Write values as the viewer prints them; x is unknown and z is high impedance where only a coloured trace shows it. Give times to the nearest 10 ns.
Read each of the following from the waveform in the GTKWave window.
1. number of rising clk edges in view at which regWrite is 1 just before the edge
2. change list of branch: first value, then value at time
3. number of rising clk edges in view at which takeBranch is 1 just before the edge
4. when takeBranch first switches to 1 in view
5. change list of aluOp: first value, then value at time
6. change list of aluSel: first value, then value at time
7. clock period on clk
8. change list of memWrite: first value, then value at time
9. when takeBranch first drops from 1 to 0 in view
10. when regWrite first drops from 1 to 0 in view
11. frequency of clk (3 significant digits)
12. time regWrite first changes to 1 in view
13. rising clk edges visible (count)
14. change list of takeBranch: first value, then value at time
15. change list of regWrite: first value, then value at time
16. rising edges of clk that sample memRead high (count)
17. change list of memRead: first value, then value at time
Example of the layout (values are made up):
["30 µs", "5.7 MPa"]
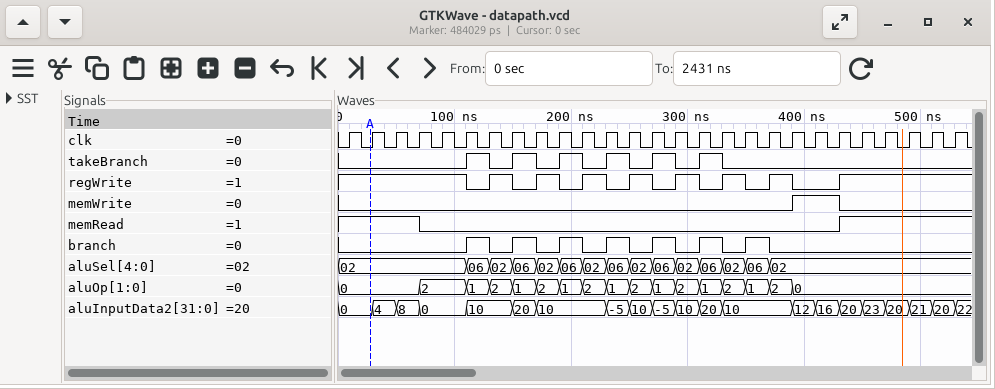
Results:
["18", "0, 1 at 110 ns, 0 at 130 ns, 1 at 150 ns, 0 at 170 ns, 1 at 190 ns, 0 at 210 ns, 1 at 230 ns, 0 at 250 ns, 1 at 270 ns, 0 at 290 ns, 1 at 310 ns, 0 at 330 ns, 1 at 350 ns, 0 at 370 ns", "6", "110 ns", "0, 2 at 70 ns, 1 at 110 ns, 2 at 130 ns, 1 at 150 ns, 2 at 170 ns, 1 at 190 ns, 2 at 210 ns, 1 at 230 ns, 2 at 250 ns, 1 at 270 ns, 2 at 290 ns, 1 at 310 ns, 2 at 330 ns, 1 at 350 ns, 2 at 370 ns, 0 at 390 ns", "02, 06 at 110 ns, 02 at 130 ns, 06 at 150 ns, 02 at 170 ns, 06 at 190 ns, 02 at 210 ns, 06 at 230 ns, 02 at 250 ns, 06 at 270 ns, 02 at 290 ns, 06 at 310 ns, 02 at 330 ns, 06 at 350 ns, 02 at 370 ns", "20 ns", "0, 1 at 390 ns, 0 at 430 ns", "130 ns", "110 ns", "50.0 MHz", "130 ns", "27", "0, 1 at 110 ns, 0 at 130 ns, 1 at 150 ns, 0 at 170 ns, 1 at 190 ns, 0 at 210 ns, 1 at 230 ns, 0 at 250 ns, 1 at 270 ns, 0 at 290 ns, 1 at 310 ns, 0 at 330 ns", "1, 0 at 110 ns, 1 at 130 ns, 0 at 150 ns, 1 at 170 ns, 0 at 190 ns, 1 at 210 ns, 0 at 230 ns, 1 at 250 ns, 0 at 270 ns, 1 at 290 ns, 0 at 310 ns, 1 at 330 ns, 0 at 350 ns, 1 at 370 ns, 0 at 390 ns, 1 at 430 ns", "9", "1, 0 at 70 ns, 1 at 430 ns"]
